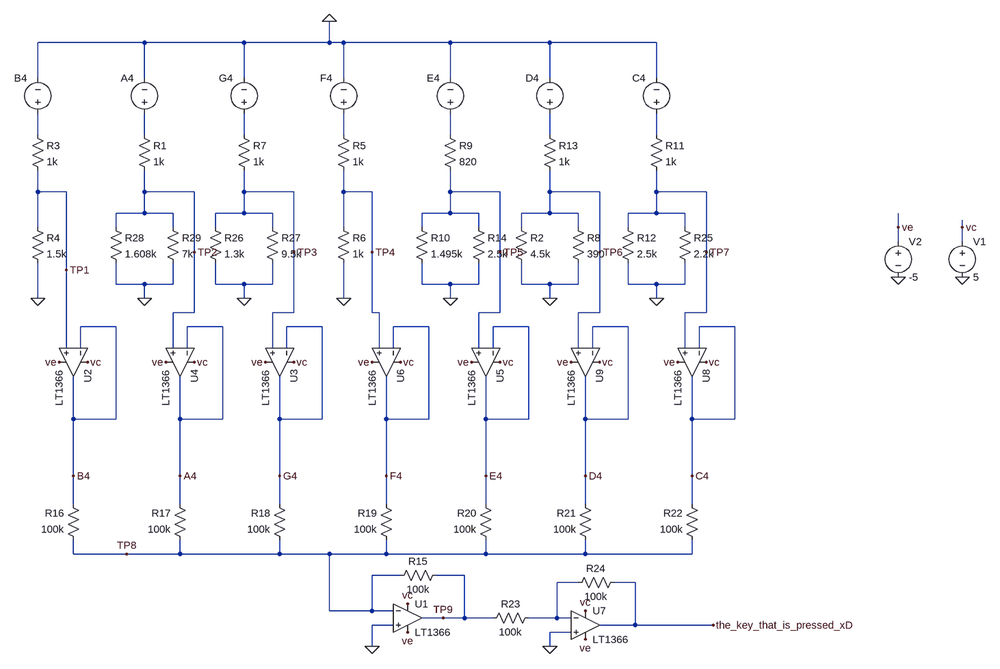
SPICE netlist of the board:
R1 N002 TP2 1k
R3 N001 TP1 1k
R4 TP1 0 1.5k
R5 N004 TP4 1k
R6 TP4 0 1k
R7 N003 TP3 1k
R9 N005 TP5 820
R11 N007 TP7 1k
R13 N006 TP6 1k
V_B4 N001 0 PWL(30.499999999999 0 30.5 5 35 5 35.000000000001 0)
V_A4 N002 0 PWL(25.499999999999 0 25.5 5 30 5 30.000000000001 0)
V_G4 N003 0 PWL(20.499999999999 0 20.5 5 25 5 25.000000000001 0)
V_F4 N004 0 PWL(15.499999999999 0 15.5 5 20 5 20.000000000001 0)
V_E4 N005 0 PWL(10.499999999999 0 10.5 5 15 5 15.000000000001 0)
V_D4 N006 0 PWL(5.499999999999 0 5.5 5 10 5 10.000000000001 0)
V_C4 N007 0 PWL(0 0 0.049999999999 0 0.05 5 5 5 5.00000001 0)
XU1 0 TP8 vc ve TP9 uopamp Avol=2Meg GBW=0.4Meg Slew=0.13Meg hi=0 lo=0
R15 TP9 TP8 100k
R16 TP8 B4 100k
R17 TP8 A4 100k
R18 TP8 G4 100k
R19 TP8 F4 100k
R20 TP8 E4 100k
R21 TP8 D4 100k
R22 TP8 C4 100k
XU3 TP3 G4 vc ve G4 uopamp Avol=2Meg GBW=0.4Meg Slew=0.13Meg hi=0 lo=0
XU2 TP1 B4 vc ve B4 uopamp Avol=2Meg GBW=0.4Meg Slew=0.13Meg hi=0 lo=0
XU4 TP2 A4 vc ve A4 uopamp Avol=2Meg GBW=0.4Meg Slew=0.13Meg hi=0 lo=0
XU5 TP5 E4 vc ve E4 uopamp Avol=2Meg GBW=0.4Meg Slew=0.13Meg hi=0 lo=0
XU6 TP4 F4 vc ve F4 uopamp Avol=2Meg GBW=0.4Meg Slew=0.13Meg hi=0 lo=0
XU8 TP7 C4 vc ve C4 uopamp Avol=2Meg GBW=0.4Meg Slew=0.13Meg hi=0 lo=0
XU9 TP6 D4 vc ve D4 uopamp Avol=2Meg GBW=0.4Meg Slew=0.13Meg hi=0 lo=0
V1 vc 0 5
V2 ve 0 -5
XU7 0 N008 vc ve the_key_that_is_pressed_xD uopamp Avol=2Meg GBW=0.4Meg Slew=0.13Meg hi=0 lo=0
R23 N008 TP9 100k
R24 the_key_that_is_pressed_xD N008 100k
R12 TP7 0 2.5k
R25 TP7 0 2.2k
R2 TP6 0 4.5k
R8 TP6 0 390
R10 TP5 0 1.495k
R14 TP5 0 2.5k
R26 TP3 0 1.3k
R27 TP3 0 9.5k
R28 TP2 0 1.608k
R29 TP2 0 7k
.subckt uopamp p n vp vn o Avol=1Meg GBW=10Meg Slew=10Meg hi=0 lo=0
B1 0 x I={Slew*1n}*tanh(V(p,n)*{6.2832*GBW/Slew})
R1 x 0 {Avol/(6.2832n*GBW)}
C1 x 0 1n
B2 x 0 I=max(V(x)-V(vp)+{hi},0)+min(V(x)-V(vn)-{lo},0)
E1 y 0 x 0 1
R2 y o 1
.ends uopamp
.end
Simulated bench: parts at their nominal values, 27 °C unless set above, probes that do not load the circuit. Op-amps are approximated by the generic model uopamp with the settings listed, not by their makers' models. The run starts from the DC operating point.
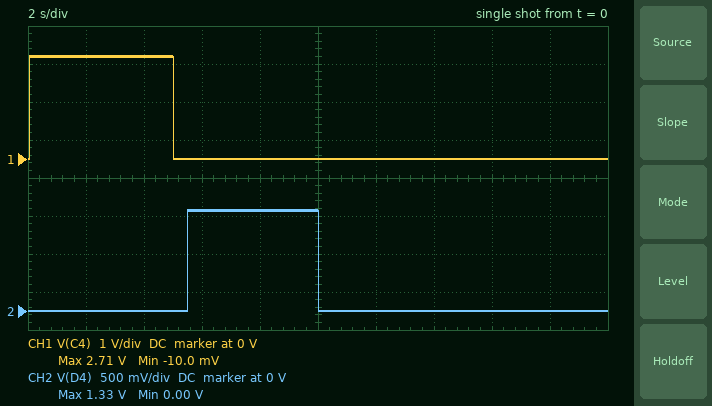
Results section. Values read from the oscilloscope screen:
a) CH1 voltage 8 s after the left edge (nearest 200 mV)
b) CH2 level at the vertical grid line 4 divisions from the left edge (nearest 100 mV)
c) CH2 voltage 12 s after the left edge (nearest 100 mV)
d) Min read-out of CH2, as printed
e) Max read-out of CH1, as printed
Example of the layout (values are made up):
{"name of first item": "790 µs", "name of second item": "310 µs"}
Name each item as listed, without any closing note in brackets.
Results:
{"CH1 voltage 8 s after the left edge": "0 V", "CH2 level at the vertical grid line 4 divisions from the left edge": "1.3 V", "CH2 voltage 12 s after the left edge": "0 V", "Min read-out of CH2, as printed": "0.00 V", "Max read-out of CH1, as printed": "2.71 V"}
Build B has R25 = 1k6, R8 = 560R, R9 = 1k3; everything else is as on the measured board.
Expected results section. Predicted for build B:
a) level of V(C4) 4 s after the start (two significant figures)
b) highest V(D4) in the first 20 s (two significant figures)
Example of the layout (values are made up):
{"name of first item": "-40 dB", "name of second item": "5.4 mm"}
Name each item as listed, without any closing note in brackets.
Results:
{"level of V(C4) 4 s after the start": "2.5 V", "highest V(D4) in the first 20 s": "1.7 V"}
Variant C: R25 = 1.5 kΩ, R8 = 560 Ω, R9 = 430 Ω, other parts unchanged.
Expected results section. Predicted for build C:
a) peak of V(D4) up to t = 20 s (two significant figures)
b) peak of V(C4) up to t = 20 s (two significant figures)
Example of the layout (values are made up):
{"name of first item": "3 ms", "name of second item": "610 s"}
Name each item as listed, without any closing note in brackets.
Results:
{"peak of V(D4) up to t = 20 s": "1.7 V", "peak of V(C4) up to t = 20 s": "2.4 V"}
